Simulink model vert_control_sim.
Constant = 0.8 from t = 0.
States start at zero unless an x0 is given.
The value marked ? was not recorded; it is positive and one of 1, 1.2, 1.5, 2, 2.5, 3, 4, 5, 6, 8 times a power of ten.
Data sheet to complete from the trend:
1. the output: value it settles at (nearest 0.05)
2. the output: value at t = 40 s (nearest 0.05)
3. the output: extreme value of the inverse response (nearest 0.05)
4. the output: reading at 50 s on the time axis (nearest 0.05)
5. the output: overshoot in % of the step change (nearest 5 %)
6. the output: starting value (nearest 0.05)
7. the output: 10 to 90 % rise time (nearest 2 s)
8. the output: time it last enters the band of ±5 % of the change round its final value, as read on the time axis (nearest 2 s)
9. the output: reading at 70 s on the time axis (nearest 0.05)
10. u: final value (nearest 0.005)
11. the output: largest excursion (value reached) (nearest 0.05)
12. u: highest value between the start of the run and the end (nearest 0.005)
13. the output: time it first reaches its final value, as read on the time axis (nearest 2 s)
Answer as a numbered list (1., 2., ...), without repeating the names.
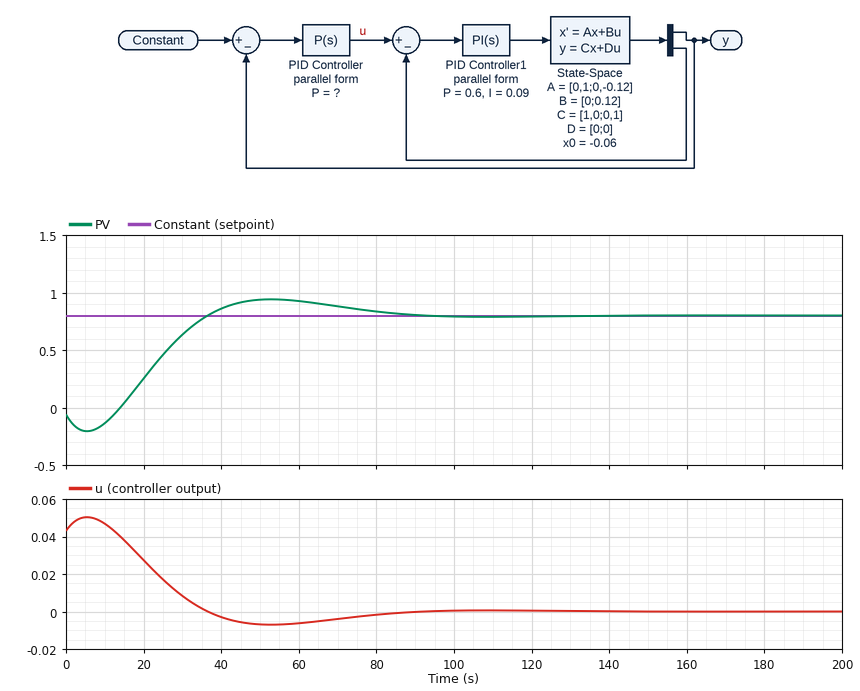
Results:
1. 0.80
2. 0.85
3. -0.20
4. 0.95
5. 15 %
6. -0.05
7. 18 s
8. 78 s
9. 0.90
10. 0.000
11. 0.95
12. 0.050
13. 36 s
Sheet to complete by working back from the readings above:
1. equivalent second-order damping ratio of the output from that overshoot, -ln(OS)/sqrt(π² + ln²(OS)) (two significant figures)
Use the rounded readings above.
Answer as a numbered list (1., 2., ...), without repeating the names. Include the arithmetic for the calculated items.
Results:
1. ln(0.15) = -1.897; 1.897 / sqrt(9.870 + 3.599) = 0.52
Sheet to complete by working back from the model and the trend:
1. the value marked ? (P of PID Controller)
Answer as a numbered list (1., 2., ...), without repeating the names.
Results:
1. 0.05
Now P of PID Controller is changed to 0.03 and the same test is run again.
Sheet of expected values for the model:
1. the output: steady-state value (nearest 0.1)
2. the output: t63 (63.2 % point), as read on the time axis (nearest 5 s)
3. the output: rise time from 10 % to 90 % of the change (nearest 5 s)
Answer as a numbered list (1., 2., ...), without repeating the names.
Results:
1. 0.8
2. 35 s
3. 30 s
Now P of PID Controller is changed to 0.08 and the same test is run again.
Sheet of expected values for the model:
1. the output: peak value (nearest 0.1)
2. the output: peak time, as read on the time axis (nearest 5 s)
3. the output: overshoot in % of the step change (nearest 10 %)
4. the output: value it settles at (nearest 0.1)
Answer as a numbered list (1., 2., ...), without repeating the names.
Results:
1. 1.1
2. 40 s
3. 30 %
4. 0.8
